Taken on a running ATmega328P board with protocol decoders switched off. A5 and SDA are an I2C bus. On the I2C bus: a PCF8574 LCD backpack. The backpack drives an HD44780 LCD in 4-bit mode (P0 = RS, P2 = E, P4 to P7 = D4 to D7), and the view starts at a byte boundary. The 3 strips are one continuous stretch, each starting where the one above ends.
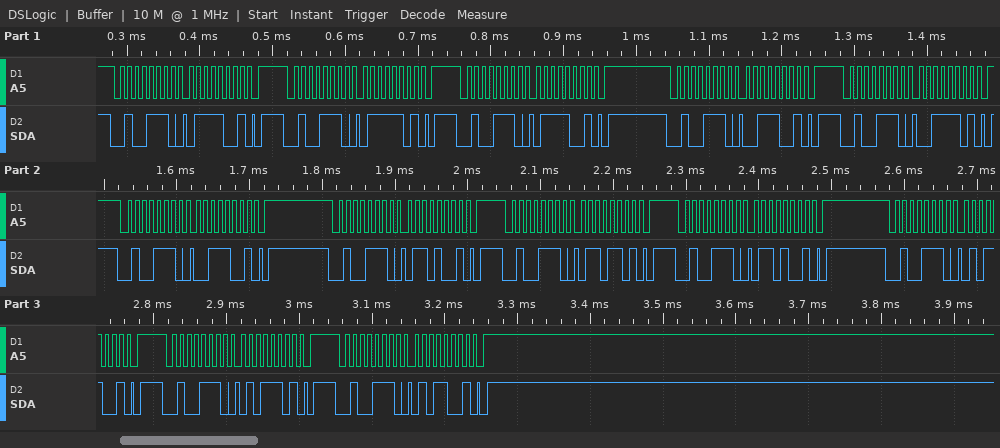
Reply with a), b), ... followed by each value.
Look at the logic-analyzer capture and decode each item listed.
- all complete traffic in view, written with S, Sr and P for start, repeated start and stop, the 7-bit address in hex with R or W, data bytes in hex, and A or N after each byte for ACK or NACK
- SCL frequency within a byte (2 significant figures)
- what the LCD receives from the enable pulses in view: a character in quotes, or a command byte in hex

a) S 27W A 79 A P S 27W A 7D A P S 27W A 79 A P S 27W A 39 A P S 27W A 3D A P S 27W A 39 A P S 27W A 69 A P S 27W A 6D A P S 27W A 69 A P S 27W A 59 A P S 27W A 5D A P S 27W A 59 A P
b) 100 kHz
c) 's' 'e'
